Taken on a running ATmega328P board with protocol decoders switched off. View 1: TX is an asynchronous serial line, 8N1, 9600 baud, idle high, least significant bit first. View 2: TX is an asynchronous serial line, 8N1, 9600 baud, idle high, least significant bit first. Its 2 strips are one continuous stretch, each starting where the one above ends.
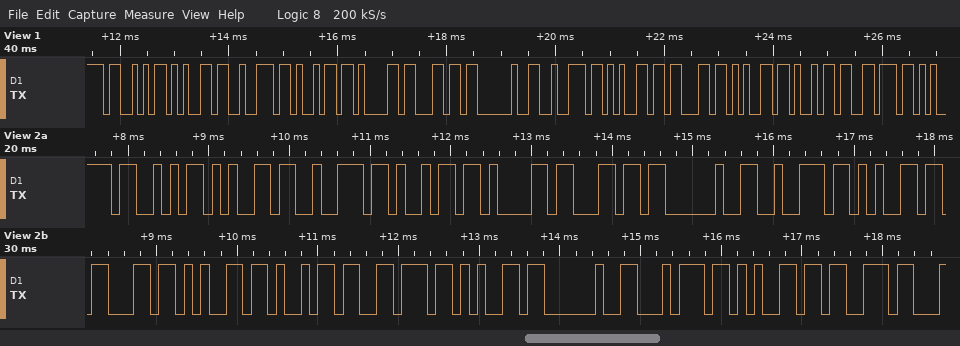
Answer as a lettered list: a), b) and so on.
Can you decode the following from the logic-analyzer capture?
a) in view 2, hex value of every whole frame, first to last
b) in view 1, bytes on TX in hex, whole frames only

a) 53 65 72 69 61 6C 20 72 65 63 65 69 76 65 20 74 65 73
b) 53 65 72 69 61 6C 20 72 65 63 65 69 76
